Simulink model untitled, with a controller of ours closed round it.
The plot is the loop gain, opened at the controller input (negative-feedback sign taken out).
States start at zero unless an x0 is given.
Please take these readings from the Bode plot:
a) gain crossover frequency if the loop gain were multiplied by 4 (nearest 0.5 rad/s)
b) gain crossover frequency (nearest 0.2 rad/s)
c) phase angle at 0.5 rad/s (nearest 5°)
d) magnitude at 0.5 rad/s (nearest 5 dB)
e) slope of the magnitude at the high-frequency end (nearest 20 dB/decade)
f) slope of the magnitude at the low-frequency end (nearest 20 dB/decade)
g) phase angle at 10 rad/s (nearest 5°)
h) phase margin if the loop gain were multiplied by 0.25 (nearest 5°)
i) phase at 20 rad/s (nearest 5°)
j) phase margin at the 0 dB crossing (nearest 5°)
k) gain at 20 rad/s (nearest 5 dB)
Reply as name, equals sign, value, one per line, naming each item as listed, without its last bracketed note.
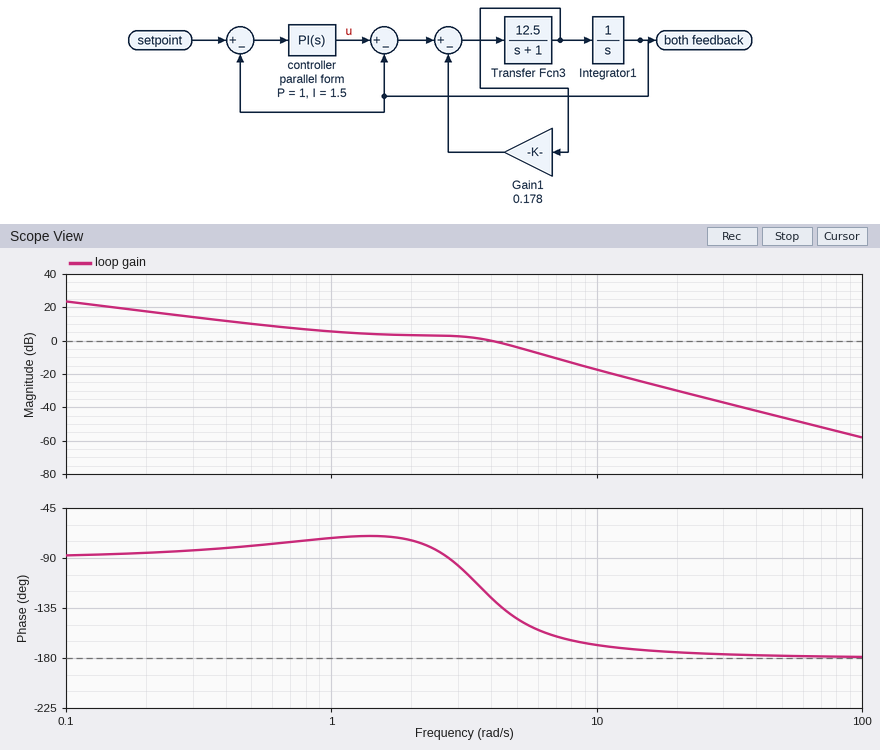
gain crossover frequency if the loop gain were multiplied by 4 = 7.5 rad/s
gain crossover frequency = 4.0 rad/s
phase angle at 0.5 rad/s = -80°
magnitude at 0.5 rad/s = 10 dB
slope of the magnitude at the high-frequency end = -40 dB/decade
slope of the magnitude at the low-frequency end = -20 dB/decade
phase angle at 10 rad/s = -170°
phase margin if the loop gain were multiplied by 0.25 = 100°
phase at 20 rad/s = -175°
phase margin at the 0 dB crossing = 55°
gain at 20 rad/s = -30 dB
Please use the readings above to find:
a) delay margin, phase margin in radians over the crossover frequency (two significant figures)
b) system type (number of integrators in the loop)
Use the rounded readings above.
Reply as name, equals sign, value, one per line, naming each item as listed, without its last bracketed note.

delay margin, phase margin in radians over the crossover frequency = 0.24 s
system type = 1
